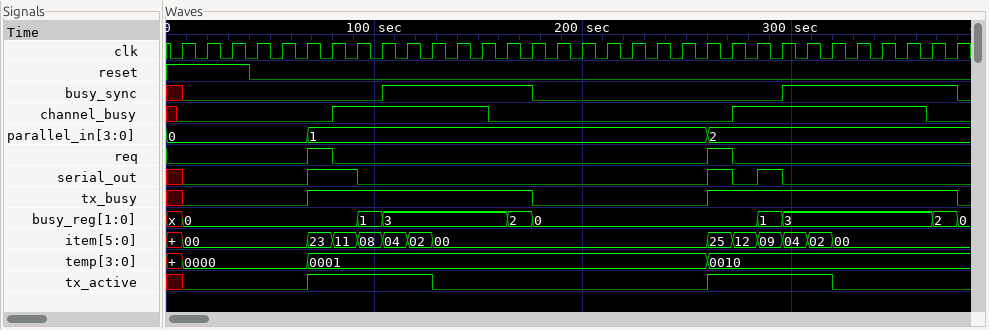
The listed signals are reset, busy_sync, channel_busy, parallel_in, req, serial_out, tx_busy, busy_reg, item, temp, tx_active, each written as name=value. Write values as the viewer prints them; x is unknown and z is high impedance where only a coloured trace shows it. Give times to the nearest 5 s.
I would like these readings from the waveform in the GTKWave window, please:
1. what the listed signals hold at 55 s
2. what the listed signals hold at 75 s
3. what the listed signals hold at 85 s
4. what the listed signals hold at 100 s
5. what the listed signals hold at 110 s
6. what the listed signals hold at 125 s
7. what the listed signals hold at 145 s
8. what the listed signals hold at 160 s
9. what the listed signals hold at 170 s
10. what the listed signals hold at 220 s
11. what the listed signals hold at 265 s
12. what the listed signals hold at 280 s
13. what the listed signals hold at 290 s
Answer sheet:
reset=0, busy_sync=0, channel_busy=0, parallel_in=0, req=0, serial_out=0, tx_busy=0, busy_reg=0, item=00, temp=0000, tx_active=0
reset=0, busy_sync=0, channel_busy=0, parallel_in=1, req=1, serial_out=1, tx_busy=1, busy_reg=0, item=23, temp=0001, tx_active=1
reset=0, busy_sync=0, channel_busy=1, parallel_in=1, req=0, serial_out=1, tx_busy=1, busy_reg=0, item=11, temp=0001, tx_active=1
reset=0, busy_sync=0, channel_busy=1, parallel_in=1, req=0, serial_out=0, tx_busy=1, busy_reg=1, item=08, temp=0001, tx_active=1
reset=0, busy_sync=1, channel_busy=1, parallel_in=1, req=0, serial_out=0, tx_busy=1, busy_reg=3, item=04, temp=0001, tx_active=1
reset=0, busy_sync=1, channel_busy=1, parallel_in=1, req=0, serial_out=0, tx_busy=1, busy_reg=3, item=02, temp=0001, tx_active=1
reset=0, busy_sync=1, channel_busy=1, parallel_in=1, req=0, serial_out=0, tx_busy=1, busy_reg=3, item=00, temp=0001, tx_active=0
reset=0, busy_sync=1, channel_busy=0, parallel_in=1, req=0, serial_out=0, tx_busy=1, busy_reg=3, item=00, temp=0001, tx_active=0
reset=0, busy_sync=1, channel_busy=0, parallel_in=1, req=0, serial_out=0, tx_busy=1, busy_reg=2, item=00, temp=0001, tx_active=0
reset=0, busy_sync=0, channel_busy=0, parallel_in=1, req=0, serial_out=0, tx_busy=0, busy_reg=0, item=00, temp=0001, tx_active=0
reset=0, busy_sync=0, channel_busy=0, parallel_in=2, req=1, serial_out=1, tx_busy=1, busy_reg=0, item=25, temp=0010, tx_active=1
reset=0, busy_sync=0, channel_busy=1, parallel_in=2, req=0, serial_out=0, tx_busy=1, busy_reg=0, item=12, temp=0010, tx_active=1
reset=0, busy_sync=0, channel_busy=1, parallel_in=2, req=0, serial_out=1, tx_busy=1, busy_reg=1, item=09, temp=0010, tx_active=1
